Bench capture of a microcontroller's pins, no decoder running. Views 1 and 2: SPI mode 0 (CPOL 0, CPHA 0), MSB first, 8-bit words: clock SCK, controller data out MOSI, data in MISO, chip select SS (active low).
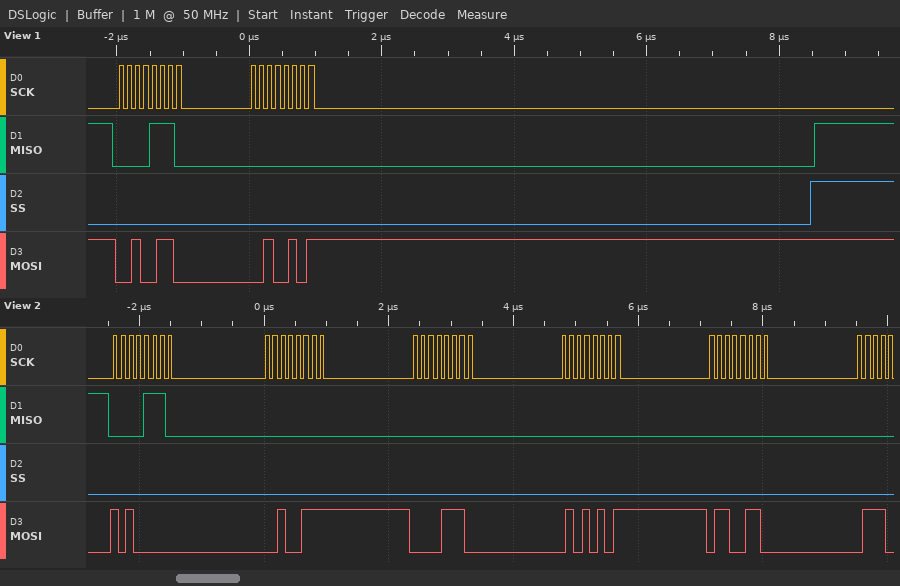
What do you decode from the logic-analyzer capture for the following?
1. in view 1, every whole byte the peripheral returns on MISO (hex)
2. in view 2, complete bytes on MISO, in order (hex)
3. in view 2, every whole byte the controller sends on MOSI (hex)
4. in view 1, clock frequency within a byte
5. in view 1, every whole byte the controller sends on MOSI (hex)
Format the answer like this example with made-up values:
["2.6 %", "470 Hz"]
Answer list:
["0E 00", "0E 00 00 00 00", "A0 27 0E 55 66", "8 MHz", "26 25"]
